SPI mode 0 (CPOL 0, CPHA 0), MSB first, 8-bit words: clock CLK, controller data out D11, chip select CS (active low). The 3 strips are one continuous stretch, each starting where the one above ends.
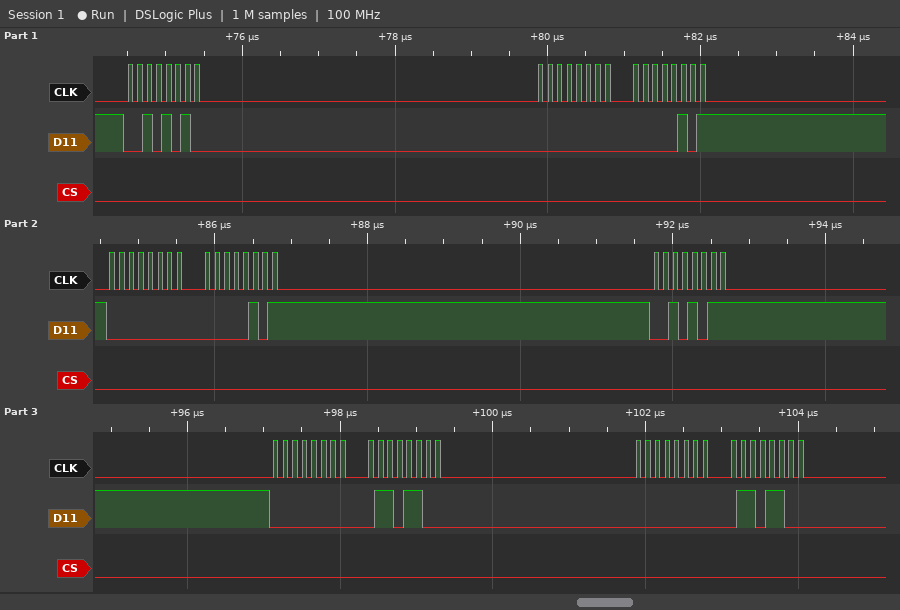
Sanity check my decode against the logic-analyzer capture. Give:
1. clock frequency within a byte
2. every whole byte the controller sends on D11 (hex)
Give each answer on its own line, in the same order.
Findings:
8 MHz
0x2A 0x00 0x05 0x00 0x05 0x2B 0x00 0x6C 0x00 0x6C
